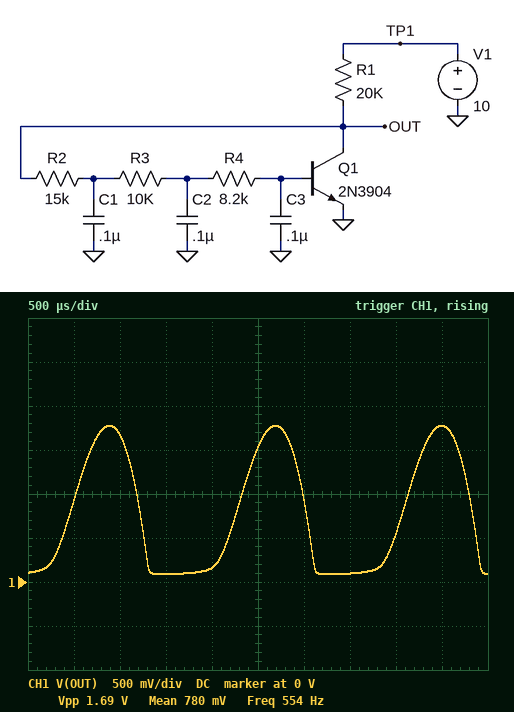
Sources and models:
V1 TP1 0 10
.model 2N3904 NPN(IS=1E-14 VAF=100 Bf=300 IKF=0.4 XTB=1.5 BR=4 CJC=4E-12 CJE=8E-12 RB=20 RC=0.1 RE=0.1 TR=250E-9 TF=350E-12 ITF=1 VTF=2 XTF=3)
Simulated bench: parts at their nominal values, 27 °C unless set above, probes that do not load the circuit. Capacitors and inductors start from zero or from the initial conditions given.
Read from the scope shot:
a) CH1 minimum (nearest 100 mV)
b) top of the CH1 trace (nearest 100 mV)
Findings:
100 mV
1.8 V
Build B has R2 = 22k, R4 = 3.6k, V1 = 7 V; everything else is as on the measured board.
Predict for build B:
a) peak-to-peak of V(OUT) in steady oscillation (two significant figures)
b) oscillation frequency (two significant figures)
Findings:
1.2 V
640 Hz
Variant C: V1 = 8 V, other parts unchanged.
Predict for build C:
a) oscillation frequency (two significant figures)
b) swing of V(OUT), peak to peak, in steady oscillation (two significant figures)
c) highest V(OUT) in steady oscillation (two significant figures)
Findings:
530 Hz
1.5 V
1.6 V
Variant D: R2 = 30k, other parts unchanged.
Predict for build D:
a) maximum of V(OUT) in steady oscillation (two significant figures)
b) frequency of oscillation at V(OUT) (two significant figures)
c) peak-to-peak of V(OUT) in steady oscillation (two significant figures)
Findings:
1.7 V
500 Hz
1.6 V
